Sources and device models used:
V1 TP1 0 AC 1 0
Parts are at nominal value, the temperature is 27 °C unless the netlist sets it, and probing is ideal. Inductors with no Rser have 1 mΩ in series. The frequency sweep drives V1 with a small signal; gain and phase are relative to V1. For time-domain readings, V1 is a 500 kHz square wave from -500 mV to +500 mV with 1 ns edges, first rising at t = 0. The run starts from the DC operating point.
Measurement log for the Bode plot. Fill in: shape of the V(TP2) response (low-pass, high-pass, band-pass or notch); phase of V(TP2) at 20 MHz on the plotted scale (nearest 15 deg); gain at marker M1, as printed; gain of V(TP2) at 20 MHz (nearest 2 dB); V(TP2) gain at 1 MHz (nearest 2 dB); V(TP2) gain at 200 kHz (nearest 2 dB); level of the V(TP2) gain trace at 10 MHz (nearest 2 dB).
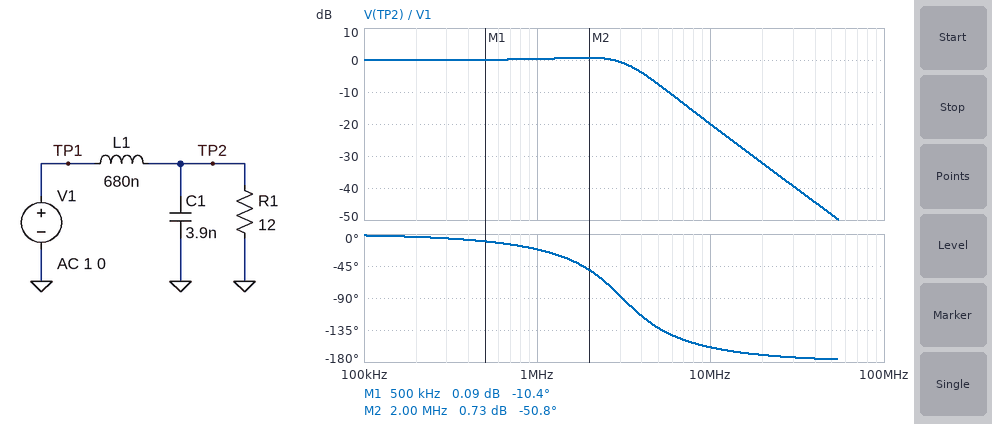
low-pass
-165 deg
0.09 dB
-32 dB
0 dB
0 dB
-20 dB
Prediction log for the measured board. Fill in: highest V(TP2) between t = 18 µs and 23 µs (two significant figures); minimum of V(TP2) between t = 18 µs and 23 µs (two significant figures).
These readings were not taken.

630 mV
-630 mV
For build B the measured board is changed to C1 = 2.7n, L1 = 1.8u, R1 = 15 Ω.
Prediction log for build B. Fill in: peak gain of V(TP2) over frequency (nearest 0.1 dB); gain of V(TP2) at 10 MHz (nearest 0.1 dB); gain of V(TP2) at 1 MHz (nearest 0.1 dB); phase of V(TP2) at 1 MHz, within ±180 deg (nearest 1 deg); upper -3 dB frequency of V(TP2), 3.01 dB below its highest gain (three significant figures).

0 dB
-25.9 dB
-0.9 dB
-43 deg
1.81 MHz
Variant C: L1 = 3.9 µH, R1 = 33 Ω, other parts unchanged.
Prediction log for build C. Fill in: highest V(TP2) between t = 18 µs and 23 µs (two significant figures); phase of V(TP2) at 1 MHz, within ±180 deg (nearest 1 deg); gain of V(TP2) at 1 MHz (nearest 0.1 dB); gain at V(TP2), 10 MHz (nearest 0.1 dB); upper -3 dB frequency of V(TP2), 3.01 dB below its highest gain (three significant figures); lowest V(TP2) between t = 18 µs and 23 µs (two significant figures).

680 mV
-62 deg
1.5 dB
-35.5 dB
1.52 MHz
-680 mV
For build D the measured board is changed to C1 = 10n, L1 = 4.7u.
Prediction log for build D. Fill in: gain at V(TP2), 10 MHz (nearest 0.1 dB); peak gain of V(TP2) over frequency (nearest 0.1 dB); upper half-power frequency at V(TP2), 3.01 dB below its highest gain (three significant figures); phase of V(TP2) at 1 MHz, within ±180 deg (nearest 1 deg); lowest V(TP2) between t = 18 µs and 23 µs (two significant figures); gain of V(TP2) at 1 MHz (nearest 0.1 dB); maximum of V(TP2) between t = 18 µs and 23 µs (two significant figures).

-45.4 dB
0 dB
545 kHz
-109 deg
-480 mV
-8.3 dB
480 mV
